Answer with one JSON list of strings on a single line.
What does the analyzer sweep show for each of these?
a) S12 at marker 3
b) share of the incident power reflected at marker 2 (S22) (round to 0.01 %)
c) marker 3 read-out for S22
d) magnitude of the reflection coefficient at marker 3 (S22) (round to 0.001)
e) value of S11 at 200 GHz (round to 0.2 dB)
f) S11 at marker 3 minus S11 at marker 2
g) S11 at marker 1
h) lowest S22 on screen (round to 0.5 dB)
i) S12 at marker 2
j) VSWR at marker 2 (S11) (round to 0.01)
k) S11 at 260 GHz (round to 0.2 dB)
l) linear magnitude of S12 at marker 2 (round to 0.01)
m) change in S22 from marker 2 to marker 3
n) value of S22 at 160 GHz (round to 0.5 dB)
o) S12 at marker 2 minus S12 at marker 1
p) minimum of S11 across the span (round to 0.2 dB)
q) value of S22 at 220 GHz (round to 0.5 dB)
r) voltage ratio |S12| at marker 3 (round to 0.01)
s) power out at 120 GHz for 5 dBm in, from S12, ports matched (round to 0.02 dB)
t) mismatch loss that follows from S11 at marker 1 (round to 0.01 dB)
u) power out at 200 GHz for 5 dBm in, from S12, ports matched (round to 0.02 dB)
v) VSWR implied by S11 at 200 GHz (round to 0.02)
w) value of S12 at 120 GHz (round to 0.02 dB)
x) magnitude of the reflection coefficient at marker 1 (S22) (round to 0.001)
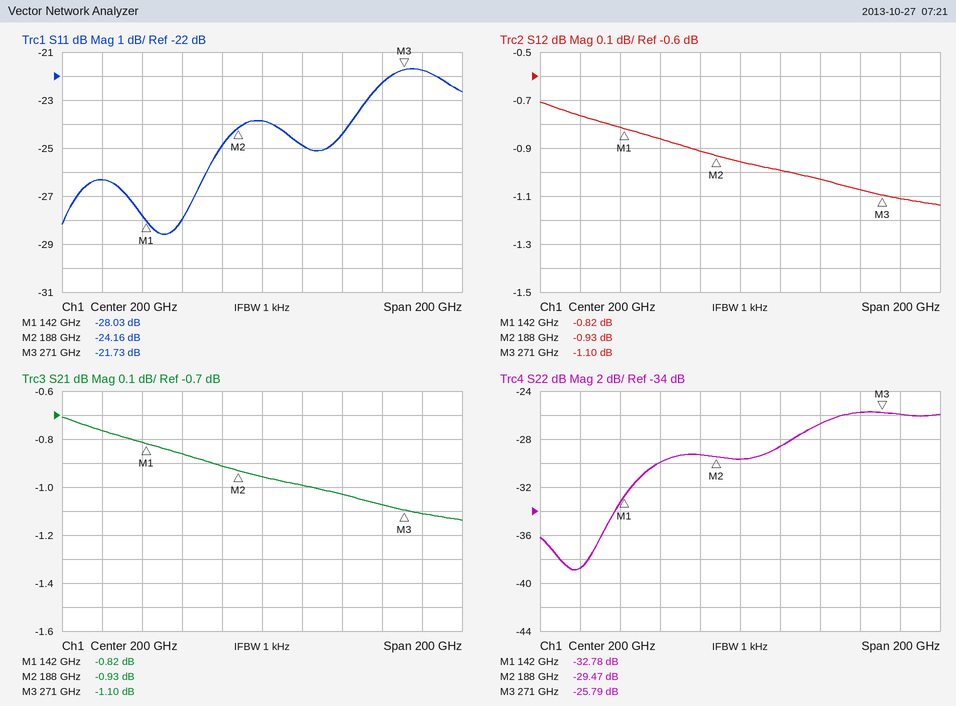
["-1.10 dB", "0.11 %", "-25.79 dB", "0.051", "-23.8 dB", "2.43 dB", "-28.03 dB", "-39.0 dB", "-0.93 dB", "1.13", "-22.2 dB", "0.90", "3.68 dB", "-30.0 dB", "-0.11 dB", "-28.6 dB", "-28.5 dB", "0.88", "4.24 dBm", "0.01 dB", "4.04 dBm", "1.14", "-0.76 dB", "0.023"]
